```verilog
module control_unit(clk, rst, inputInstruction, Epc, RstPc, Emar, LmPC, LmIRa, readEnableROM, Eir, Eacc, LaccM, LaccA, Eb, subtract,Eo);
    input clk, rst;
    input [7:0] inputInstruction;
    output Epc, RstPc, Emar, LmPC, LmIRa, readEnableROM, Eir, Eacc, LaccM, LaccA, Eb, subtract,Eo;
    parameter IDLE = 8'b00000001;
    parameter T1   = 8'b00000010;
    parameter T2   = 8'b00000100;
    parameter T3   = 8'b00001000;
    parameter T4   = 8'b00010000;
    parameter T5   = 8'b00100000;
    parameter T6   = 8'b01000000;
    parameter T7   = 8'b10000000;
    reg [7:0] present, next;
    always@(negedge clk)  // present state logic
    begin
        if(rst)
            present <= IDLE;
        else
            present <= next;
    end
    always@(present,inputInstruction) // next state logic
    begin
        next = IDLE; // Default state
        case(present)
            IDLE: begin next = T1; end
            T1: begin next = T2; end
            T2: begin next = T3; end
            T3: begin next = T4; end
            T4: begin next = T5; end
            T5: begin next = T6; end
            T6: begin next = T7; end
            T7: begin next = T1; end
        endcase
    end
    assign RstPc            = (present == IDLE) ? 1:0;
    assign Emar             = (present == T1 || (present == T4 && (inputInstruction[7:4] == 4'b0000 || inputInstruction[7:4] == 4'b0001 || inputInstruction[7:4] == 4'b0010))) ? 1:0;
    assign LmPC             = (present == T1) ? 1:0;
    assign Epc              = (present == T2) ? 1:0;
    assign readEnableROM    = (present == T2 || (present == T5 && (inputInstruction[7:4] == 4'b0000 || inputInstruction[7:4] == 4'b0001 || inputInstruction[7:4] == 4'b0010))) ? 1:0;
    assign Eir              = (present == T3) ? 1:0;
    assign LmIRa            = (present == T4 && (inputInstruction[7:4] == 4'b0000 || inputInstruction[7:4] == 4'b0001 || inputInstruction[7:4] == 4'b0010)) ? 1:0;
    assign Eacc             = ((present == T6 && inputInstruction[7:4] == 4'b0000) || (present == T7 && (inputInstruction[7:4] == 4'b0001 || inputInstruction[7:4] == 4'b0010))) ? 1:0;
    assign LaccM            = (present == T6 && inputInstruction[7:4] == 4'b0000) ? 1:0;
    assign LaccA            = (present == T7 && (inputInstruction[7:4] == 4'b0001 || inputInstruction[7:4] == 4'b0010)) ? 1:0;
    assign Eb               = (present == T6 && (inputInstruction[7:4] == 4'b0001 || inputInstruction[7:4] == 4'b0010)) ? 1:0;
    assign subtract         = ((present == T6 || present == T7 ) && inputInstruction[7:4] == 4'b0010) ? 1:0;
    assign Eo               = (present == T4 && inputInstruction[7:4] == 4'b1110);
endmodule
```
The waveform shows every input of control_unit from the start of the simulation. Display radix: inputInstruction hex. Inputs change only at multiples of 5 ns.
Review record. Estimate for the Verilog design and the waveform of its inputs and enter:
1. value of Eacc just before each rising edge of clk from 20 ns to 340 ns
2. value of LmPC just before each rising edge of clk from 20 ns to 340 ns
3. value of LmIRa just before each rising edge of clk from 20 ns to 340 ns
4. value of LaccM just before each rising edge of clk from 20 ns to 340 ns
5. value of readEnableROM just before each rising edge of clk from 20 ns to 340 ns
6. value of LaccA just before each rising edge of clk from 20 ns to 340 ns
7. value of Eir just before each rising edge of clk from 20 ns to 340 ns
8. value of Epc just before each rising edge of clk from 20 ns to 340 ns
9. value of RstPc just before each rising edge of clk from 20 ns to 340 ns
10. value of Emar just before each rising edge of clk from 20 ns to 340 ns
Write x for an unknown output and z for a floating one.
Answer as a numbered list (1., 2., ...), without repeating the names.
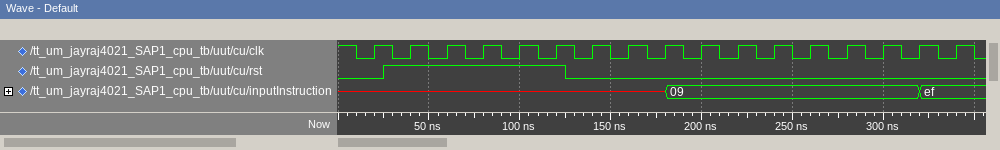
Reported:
1. x 0 0 0 0 0 0 0 0 0 0 1 0 0 0 0 0
2. x 0 0 0 0 0 1 0 0 0 0 0 0 1 0 0 0
3. x 0 0 0 0 0 0 0 0 1 0 0 0 0 0 0 0
4. x 0 0 0 0 0 0 0 0 0 0 1 0 0 0 0 0
5. x 0 0 0 0 0 0 1 0 0 1 0 0 0 1 0 0
6. x 0 0 0 0 0 0 0 0 0 0 0 0 0 0 0 0
7. x 0 0 0 0 0 0 0 1 0 0 0 0 0 0 1 0
8. x 0 0 0 0 0 0 1 0 0 0 0 0 0 1 0 0
9. x 1 1 1 1 1 0 0 0 0 0 0 0 0 0 0 0
10. x 0 0 0 0 0 1 0 0 1 0 0 0 1 0 0 0
